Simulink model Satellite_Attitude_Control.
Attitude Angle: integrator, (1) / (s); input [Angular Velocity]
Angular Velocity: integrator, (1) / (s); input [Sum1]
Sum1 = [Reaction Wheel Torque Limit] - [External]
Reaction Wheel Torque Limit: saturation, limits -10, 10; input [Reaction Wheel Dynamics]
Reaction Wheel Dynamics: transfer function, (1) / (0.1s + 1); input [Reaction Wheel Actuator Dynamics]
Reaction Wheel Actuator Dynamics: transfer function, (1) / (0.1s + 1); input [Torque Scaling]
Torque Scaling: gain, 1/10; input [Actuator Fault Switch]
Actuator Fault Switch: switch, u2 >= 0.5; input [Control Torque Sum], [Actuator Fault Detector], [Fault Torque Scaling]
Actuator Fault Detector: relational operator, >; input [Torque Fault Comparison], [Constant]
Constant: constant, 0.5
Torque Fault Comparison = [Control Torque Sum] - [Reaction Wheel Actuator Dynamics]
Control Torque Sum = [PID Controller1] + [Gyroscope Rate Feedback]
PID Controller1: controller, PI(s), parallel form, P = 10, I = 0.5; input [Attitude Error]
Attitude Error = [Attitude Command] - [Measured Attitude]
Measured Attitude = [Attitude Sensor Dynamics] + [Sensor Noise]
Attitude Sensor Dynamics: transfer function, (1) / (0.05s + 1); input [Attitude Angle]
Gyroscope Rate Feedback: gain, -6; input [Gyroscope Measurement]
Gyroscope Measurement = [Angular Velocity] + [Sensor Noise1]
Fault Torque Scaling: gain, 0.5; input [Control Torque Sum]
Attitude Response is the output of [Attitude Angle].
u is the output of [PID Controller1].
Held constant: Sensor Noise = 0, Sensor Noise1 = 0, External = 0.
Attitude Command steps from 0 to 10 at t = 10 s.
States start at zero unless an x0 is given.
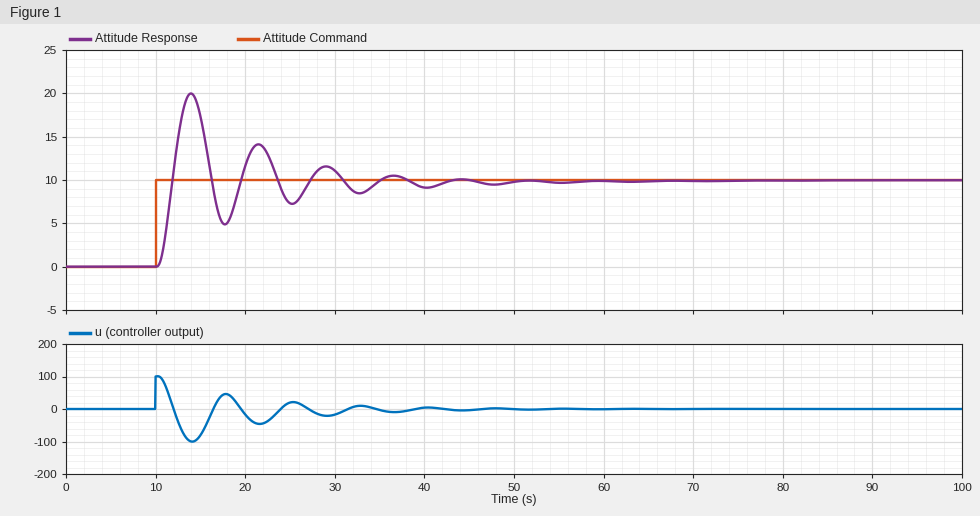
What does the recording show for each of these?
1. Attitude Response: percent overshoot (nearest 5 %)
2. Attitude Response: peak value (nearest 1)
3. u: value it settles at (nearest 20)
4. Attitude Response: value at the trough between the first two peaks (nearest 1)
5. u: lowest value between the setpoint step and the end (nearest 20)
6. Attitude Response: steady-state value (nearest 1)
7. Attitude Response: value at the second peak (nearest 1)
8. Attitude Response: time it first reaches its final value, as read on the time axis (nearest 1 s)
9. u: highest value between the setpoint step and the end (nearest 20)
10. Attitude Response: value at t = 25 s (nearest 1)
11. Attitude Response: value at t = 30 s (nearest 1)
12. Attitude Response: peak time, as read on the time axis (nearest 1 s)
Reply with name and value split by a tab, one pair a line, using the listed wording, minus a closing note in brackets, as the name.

Attitude Response: percent overshoot	100 %
Attitude Response: peak value	20
u: value it settles at	0
Attitude Response: value at the trough between the first two peaks	5
u: lowest value between the setpoint step and the end	-100
Attitude Response: steady-state value	10
Attitude Response: value at the second peak	14
Attitude Response: time it first reaches its final value, as read on the time axis	12 s
u: highest value between the setpoint step and the end	100
Attitude Response: value at t = 25 s	7
Attitude Response: value at t = 30 s	11
Attitude Response: peak time, as read on the time axis	14 s
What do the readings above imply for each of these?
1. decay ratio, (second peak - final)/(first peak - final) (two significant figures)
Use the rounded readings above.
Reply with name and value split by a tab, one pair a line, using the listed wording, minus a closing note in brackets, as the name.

decay ratio, (second peak - final)/(first peak - final)	0.40
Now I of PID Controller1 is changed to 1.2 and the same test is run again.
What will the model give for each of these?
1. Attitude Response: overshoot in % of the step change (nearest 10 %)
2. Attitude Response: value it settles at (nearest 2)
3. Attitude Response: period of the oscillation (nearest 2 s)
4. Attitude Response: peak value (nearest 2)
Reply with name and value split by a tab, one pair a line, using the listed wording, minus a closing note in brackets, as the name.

Attitude Response: overshoot in % of the step change	110 %
Attitude Response: value it settles at	10
Attitude Response: period of the oscillation	8 s
Attitude Response: peak value	22
